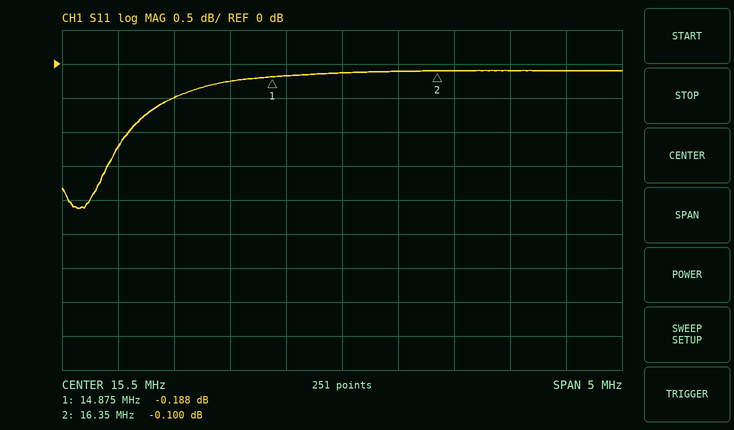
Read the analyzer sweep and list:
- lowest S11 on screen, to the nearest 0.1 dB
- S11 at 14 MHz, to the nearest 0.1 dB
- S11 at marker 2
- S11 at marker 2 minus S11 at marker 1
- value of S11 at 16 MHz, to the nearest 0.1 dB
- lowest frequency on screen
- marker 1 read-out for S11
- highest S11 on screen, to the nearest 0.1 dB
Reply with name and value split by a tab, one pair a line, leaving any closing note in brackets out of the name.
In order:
lowest S11 on screen, to the nearest 0.1 dB	-2.1 dB
S11 at 14 MHz, to the nearest 0.1 dB	-0.5 dB
S11 at marker 2	-0.100 dB
S11 at marker 2 minus S11 at marker 1	0.088 dB
value of S11 at 16 MHz, to the nearest 0.1 dB	-0.1 dB
lowest frequency on screen	13 MHz
marker 1 read-out for S11	-0.188 dB
highest S11 on screen, to the nearest 0.1 dB	-0.1 dB
